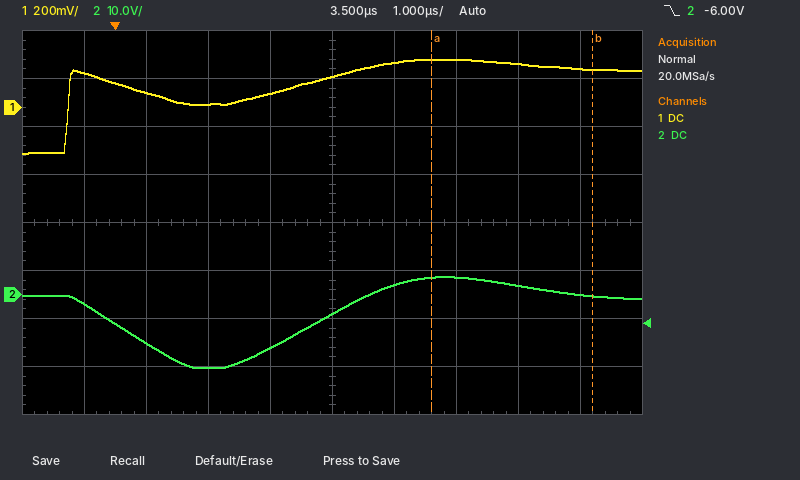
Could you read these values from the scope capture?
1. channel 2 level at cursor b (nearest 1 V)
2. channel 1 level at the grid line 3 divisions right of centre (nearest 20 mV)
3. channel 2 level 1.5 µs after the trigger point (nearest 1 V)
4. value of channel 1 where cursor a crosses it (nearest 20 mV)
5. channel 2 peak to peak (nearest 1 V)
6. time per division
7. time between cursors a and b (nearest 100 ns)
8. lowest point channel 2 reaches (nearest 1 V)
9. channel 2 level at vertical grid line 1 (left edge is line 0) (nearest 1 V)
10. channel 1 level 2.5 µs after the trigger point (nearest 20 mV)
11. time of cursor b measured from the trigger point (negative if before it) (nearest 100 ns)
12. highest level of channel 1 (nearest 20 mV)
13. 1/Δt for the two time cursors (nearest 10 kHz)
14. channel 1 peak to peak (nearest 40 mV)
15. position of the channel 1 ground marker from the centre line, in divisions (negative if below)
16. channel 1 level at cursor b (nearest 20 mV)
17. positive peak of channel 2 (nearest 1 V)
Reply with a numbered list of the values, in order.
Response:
1. 0 V
2. 180 mV
3. -15 V
4. 200 mV
5. 19 V
6. 1 µs
7. 2.6 µs
8. -15 V
9. -2 V
10. 60 mV
11. +7.7 µs
12. 200 mV
13. 380 kHz
14. 400 mV
15. +2.4 div
16. 160 mV
17. 4 V
